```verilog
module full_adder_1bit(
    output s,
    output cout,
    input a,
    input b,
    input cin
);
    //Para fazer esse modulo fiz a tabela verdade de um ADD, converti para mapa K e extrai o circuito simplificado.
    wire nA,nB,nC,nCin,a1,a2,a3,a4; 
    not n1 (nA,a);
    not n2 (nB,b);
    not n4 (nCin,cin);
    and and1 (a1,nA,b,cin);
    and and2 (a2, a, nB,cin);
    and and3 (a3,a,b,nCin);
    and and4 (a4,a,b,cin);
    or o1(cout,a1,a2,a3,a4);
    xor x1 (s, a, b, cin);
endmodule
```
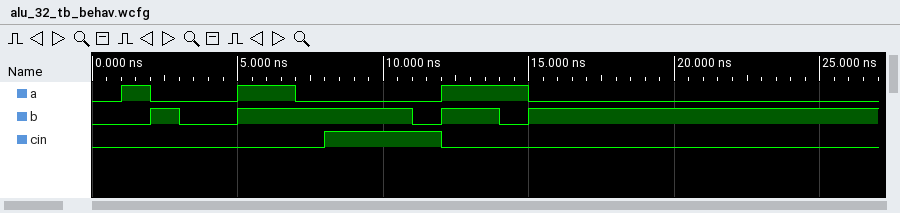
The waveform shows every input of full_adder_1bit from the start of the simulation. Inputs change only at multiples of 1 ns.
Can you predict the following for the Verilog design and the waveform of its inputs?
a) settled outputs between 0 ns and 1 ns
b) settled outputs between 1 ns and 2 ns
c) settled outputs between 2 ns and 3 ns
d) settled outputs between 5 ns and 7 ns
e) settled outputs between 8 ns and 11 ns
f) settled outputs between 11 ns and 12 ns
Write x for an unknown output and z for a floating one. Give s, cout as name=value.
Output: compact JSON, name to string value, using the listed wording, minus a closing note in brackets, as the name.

{"settled outputs between 0 ns and 1 ns": "s=0, cout=0", "settled outputs between 1 ns and 2 ns": "s=1, cout=0", "settled outputs between 2 ns and 3 ns": "s=1, cout=0", "settled outputs between 5 ns and 7 ns": "s=0, cout=1", "settled outputs between 8 ns and 11 ns": "s=0, cout=1", "settled outputs between 11 ns and 12 ns": "s=1, cout=0"}
